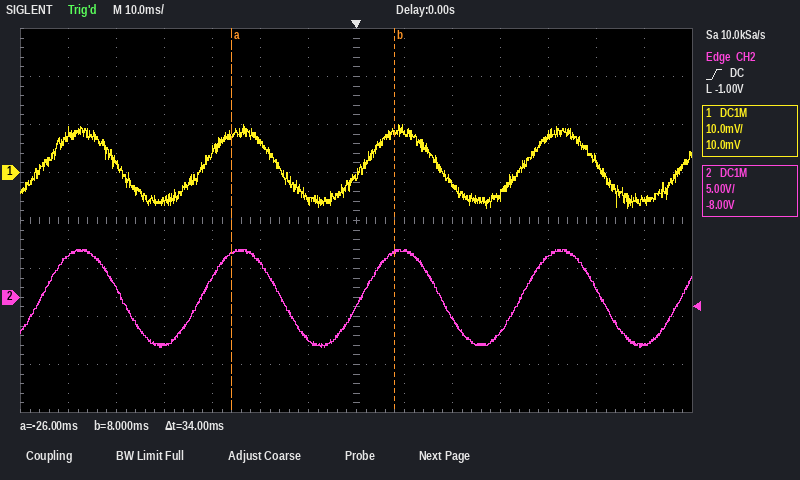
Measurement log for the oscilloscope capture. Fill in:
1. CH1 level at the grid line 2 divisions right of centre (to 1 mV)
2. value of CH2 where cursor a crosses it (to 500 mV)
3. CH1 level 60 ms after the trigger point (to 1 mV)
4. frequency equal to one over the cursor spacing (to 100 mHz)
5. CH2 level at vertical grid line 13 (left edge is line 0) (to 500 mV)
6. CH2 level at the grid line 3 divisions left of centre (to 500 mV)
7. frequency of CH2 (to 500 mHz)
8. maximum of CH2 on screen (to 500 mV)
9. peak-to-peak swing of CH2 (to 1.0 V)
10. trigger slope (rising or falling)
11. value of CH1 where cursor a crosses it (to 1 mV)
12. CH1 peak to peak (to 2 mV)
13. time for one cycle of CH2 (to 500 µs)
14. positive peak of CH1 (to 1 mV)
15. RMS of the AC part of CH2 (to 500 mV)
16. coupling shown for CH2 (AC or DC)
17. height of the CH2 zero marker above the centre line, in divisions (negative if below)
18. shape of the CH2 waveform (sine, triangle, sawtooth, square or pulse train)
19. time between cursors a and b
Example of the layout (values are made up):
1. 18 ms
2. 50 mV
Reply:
1. -2 mV
2. 4.5 V
3. -6 mV
4. 29.4 Hz
5. -5.0 V
6. 2.0 V
7. 30.0 Hz
8. 5.0 V
9. 10.0 V
10. rising
11. 8 mV
12. 18 mV
13. 33.5 ms
14. 10 mV
15. 3.5 V
16. DC
17. -1.6 div
18. sine
19. 34 ms
